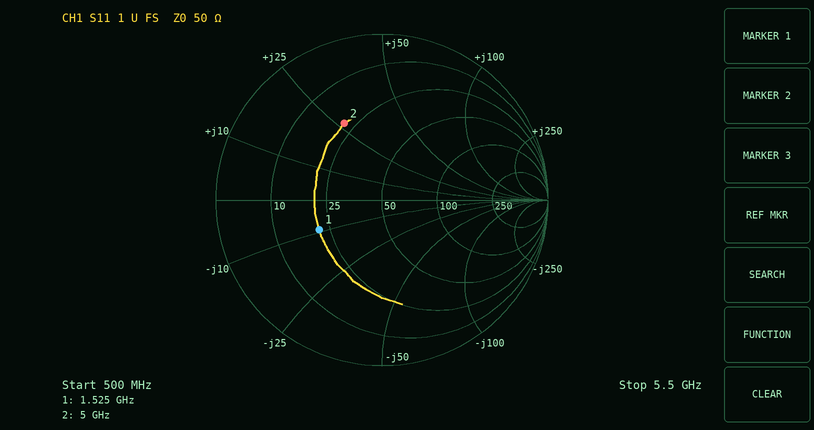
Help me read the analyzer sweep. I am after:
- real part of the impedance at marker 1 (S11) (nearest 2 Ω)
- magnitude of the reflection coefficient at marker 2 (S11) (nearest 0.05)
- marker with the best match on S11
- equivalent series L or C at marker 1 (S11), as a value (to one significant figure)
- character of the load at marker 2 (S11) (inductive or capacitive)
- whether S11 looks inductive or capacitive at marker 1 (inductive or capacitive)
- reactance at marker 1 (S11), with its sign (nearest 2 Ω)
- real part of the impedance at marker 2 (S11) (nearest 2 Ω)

22 Ω
0.50
marker 1
10 pF
inductive
capacitive
-10 Ω
22 Ω
